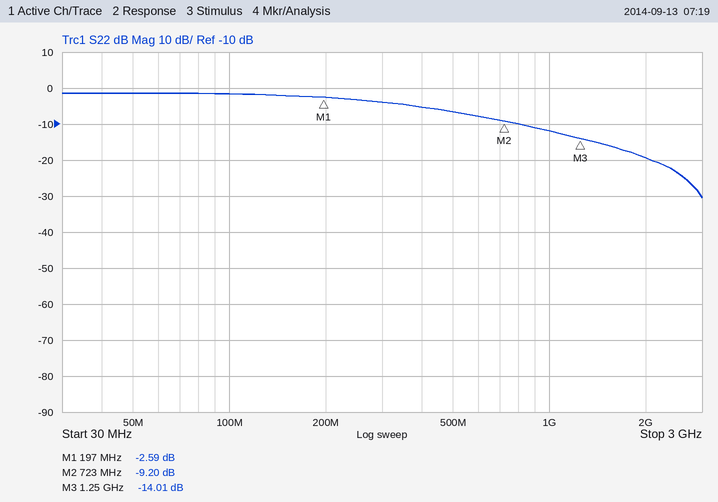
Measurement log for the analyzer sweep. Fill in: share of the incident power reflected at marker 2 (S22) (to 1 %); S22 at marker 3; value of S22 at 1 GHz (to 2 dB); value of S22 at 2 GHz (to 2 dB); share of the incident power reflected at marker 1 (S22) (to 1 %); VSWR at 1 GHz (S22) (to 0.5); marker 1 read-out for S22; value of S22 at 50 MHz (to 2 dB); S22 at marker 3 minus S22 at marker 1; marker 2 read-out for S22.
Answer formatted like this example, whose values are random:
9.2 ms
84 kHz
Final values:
12 %
-14.01 dB
-12 dB
-20 dB
55 %
1.5
-2.59 dB
-2 dB
-11.42 dB
-9.20 dB
